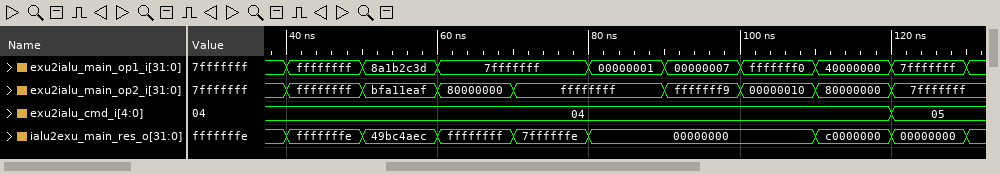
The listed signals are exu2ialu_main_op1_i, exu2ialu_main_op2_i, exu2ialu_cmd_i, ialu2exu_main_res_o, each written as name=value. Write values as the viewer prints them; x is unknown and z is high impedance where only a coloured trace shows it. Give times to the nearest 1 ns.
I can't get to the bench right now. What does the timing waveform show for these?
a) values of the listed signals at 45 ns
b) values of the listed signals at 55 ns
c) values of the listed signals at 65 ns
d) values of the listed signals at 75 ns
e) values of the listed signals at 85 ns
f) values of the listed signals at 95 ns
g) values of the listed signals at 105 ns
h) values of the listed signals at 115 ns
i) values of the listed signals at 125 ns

exu2ialu_main_op1_i=ffffffff, exu2ialu_main_op2_i=ffffffff, exu2ialu_cmd_i=04, ialu2exu_main_res_o=fffffffe
exu2ialu_main_op1_i=8a1b2c3d, exu2ialu_main_op2_i=bfa11eaf, exu2ialu_cmd_i=04, ialu2exu_main_res_o=49bc4aec
exu2ialu_main_op1_i=7fffffff, exu2ialu_main_op2_i=80000000, exu2ialu_cmd_i=04, ialu2exu_main_res_o=ffffffff
exu2ialu_main_op1_i=7fffffff, exu2ialu_main_op2_i=ffffffff, exu2ialu_cmd_i=04, ialu2exu_main_res_o=7ffffffe
exu2ialu_main_op1_i=00000001, exu2ialu_main_op2_i=ffffffff, exu2ialu_cmd_i=04, ialu2exu_main_res_o=00000000
exu2ialu_main_op1_i=00000007, exu2ialu_main_op2_i=fffffff9, exu2ialu_cmd_i=04, ialu2exu_main_res_o=00000000
exu2ialu_main_op1_i=fffffff0, exu2ialu_main_op2_i=00000010, exu2ialu_cmd_i=04, ialu2exu_main_res_o=00000000
exu2ialu_main_op1_i=40000000, exu2ialu_main_op2_i=80000000, exu2ialu_cmd_i=04, ialu2exu_main_res_o=c0000000
exu2ialu_main_op1_i=7fffffff, exu2ialu_main_op2_i=7fffffff, exu2ialu_cmd_i=05, ialu2exu_main_res_o=00000000
